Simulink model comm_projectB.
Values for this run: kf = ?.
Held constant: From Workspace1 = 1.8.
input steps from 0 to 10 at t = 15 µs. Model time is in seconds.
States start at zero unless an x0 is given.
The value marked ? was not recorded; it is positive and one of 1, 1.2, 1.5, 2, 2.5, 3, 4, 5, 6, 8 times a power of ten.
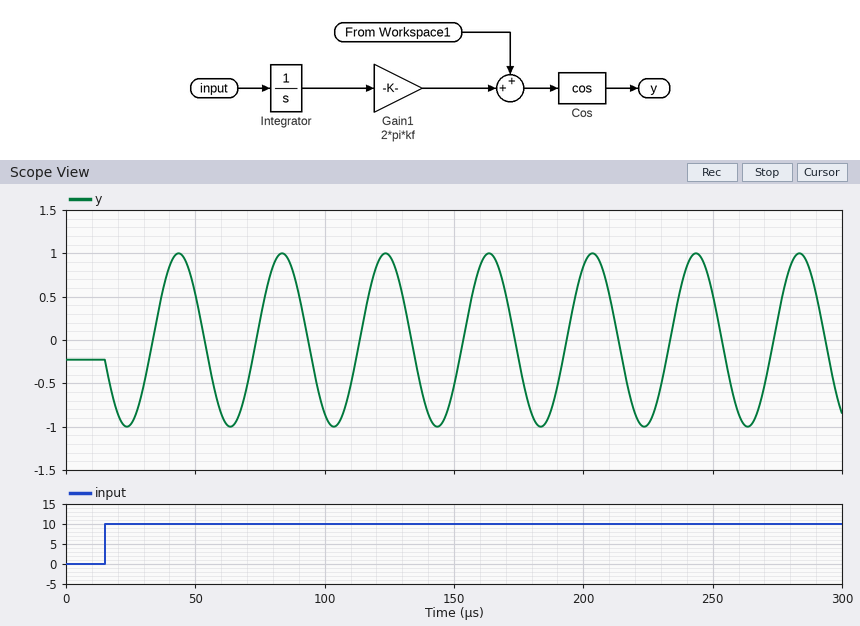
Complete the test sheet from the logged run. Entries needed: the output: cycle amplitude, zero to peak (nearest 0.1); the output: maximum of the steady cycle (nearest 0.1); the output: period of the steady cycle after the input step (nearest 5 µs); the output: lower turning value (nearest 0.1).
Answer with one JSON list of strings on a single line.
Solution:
["1.0", "1.0", "40 µs", "-1.0"]
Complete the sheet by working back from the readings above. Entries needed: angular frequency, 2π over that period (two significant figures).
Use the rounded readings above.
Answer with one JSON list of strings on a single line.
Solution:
["0.16 rad/µs"]
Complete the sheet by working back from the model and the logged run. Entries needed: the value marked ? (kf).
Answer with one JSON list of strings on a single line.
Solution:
["2500"]
